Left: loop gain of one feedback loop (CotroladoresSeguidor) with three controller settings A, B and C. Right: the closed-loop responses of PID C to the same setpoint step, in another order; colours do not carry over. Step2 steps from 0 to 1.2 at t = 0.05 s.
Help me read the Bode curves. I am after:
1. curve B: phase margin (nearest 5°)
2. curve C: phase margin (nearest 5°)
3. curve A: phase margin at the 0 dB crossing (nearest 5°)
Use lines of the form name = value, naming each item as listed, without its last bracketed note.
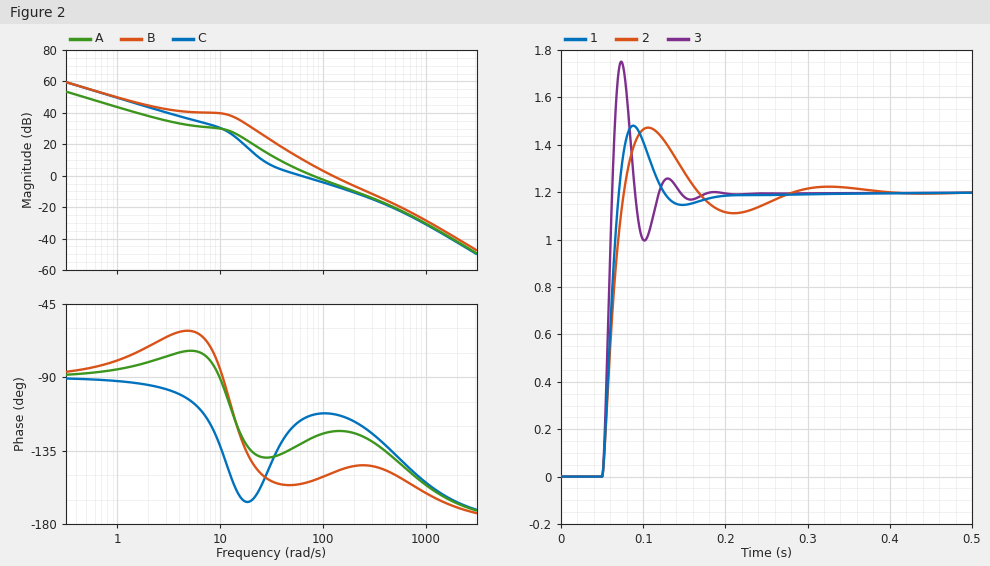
curve B: phase margin = 30°
curve C: phase margin = 65°
curve A: phase margin at the 0 dB crossing = 55°
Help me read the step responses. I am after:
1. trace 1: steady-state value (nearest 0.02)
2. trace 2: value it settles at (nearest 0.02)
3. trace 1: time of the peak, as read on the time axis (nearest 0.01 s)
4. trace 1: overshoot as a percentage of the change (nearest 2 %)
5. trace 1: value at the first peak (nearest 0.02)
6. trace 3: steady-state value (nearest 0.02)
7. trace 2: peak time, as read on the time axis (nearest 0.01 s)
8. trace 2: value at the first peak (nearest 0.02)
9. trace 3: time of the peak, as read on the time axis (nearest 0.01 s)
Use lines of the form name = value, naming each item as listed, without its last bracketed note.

trace 1: steady-state value = 1.20
trace 2: value it settles at = 1.20
trace 1: time of the peak, as read on the time axis = 0.09 s
trace 1: overshoot as a percentage of the change = 24 %
trace 1: value at the first peak = 1.48
trace 3: steady-state value = 1.20
trace 2: peak time, as read on the time axis = 0.11 s
trace 2: value at the first peak = 1.48
trace 3: time of the peak, as read on the time axis = 0.07 s
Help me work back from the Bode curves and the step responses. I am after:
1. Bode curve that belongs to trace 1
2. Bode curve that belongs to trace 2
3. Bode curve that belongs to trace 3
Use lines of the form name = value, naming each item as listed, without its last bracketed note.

Bode curve that belongs to trace 1 = A
Bode curve that belongs to trace 2 = C
Bode curve that belongs to trace 3 = B
